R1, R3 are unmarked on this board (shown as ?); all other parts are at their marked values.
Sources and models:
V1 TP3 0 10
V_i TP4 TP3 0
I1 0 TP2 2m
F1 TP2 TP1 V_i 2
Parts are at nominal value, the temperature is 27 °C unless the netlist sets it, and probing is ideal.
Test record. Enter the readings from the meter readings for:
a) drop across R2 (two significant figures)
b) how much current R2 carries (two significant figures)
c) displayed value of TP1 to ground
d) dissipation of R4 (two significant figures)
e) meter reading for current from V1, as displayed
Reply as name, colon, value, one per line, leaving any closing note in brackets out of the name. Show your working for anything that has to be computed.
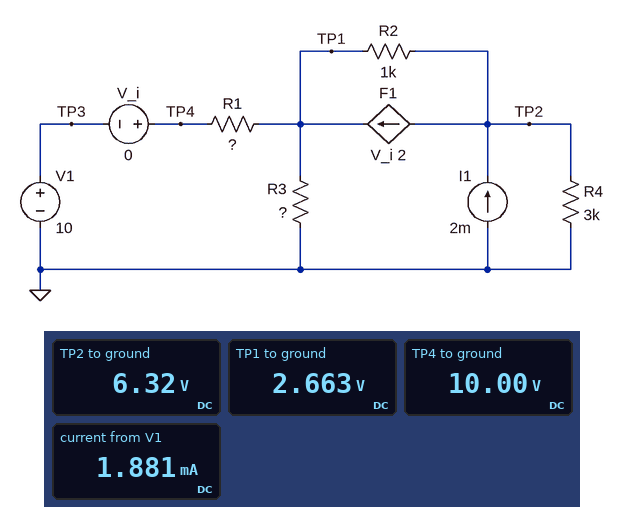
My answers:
drop across R2: 6.32 V - 2.663 V = 3.7 V
how much current R2 carries: (6.32 V - 2.663 V) / 1 kΩ = 3.7 mA
displayed value of TP1 to ground: 2.663 V
dissipation of R4: (6.32 V)^2 / 3 kΩ = 13 mW
meter reading for current from V1, as displayed: 1.881 mA
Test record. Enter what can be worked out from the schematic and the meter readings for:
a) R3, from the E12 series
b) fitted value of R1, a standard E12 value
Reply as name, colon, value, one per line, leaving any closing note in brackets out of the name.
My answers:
R3, from the E12 series: 1.5 kΩ
fitted value of R1, a standard E12 value: 3.9 kΩ
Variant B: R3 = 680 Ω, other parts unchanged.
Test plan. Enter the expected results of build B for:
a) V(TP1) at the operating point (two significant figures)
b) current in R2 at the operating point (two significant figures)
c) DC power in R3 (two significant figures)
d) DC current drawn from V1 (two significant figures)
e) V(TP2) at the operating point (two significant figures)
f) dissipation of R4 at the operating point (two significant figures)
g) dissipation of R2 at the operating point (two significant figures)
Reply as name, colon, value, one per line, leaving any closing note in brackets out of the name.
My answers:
V(TP1) at the operating point: 1.5 V
current in R2 at the operating point: 4.4 mA
DC power in R3: 3.3 mW
DC current drawn from V1: 2.2 mA
V(TP2) at the operating point: 5.9 V
dissipation of R4 at the operating point: 12 mW
dissipation of R2 at the operating point: 19 mW
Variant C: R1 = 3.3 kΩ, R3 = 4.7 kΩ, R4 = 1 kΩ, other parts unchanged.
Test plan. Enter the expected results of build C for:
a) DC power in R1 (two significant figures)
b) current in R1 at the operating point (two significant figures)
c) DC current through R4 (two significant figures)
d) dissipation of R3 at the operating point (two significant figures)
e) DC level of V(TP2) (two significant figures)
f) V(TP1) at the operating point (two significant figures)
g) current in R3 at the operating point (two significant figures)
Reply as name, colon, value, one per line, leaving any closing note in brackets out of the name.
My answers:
DC power in R1: 22 mW
current in R1 at the operating point: 2.6 mA
DC current through R4: 4.3 mA
dissipation of R3 at the operating point: 420 µW
DC level of V(TP2): 4.3 V
V(TP1) at the operating point: 1.4 V
current in R3 at the operating point: 300 µA
